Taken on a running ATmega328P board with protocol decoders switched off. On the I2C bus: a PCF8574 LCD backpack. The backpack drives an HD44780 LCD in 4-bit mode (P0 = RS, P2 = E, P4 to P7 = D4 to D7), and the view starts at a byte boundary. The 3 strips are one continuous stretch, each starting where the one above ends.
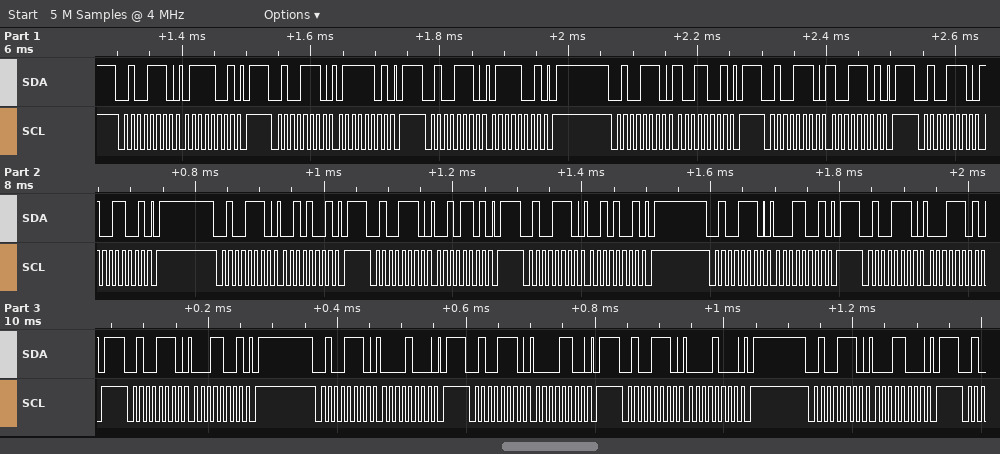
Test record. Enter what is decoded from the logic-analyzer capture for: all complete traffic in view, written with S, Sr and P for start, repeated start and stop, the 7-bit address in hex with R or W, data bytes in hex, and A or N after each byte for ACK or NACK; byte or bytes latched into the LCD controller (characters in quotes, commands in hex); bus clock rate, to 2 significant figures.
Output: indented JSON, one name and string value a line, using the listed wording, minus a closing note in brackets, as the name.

{
  "all complete traffic in view, written with S, Sr and P for start, repeated start and stop, the 7-bit address in hex with R or W, data bytes in hex, and A or N after each byte for ACK or NACK": "S 27W A 79 A P S 27W A 7D A P S 27W A 79 A P S 27W A 99 A P S 27W A 9D A P S 27W A 99 A P S 27W A 29 A P S 27W A 2D A P S 27W A 29 A P S 27W A 19 A P S 27W A 1D A P S 27W A 19 A P S 27W A 08 A P S 27W A 0C A P S 27W A 08 A P S 27W A 18 A P",
  "byte or bytes latched into the LCD controller": "'y' '!'",
  "bus clock rate, to 2 significant figures": "100 kHz"
}
